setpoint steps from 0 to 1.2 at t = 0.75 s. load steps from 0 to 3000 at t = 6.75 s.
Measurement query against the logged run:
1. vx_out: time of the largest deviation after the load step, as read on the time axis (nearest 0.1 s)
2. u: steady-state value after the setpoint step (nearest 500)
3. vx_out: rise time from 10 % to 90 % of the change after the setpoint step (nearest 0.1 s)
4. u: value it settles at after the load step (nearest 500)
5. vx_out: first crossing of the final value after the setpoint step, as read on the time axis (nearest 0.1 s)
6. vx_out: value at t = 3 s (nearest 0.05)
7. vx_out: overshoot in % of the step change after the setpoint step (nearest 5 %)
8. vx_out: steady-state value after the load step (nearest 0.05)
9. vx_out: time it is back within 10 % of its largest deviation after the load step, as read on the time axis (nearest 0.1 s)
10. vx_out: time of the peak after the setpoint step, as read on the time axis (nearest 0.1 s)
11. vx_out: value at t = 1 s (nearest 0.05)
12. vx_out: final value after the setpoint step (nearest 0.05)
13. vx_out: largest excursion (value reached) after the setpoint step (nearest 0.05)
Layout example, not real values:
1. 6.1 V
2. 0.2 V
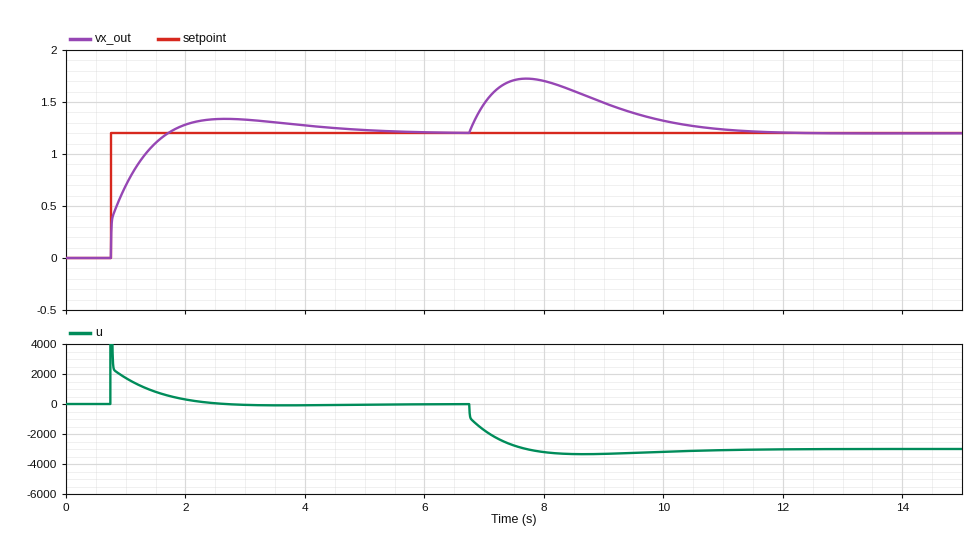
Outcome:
1. 7.7 s
2. 0
3. 0.7 s
4. -3000
5. 1.7 s
6. 1.35
7. 10 %
8. 1.20
9. 10.7 s
10. 2.7 s
11. 0.70
12. 1.20
13. 1.35
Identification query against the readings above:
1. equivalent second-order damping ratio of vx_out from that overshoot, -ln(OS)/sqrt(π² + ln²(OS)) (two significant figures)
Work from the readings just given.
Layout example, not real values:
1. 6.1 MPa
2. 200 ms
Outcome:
1. 0.59
